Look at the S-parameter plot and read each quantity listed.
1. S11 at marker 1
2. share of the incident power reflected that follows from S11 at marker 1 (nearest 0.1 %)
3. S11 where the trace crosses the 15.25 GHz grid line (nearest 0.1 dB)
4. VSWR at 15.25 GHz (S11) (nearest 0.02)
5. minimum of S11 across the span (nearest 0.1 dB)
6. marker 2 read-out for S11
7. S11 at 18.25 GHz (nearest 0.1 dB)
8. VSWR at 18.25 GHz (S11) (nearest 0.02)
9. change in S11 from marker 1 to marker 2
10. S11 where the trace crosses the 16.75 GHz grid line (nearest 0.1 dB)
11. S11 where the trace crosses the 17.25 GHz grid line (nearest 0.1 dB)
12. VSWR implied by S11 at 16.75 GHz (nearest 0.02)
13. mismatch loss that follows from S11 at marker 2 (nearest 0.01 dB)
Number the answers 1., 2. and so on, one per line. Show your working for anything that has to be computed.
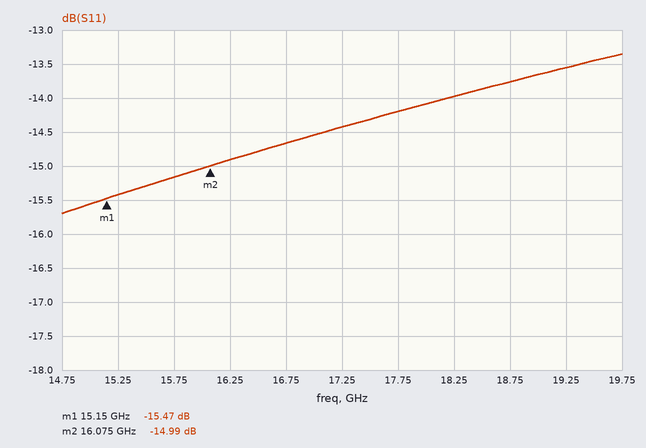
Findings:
1. -15.47 dB
2. 10^(-15.47/10) ≈ 2.8 %
3. -15.4 dB
4. |Γ| = 10^(-15.4/20) = 0.1698; VSWR = (1 + 0.1698)/(1 − 0.1698) ≈ 1.41, so 1.40 to the nearest 0.02
5. -15.7 dB
6. -14.99 dB
7. -14.0 dB
8. |Γ| = 10^(-14/20) = 0.1995; VSWR = (1 + 0.1995)/(1 − 0.1995) ≈ 1.50
9. -14.99 − (-15.47) = 0.48 dB
10. -14.7 dB
11. -14.4 dB
12. |Γ| = 10^(-14.7/20) = 0.1841; VSWR = (1 + 0.1841)/(1 − 0.1841) ≈ 1.45, so 1.46 to the nearest 0.02
13. −10 log10(1 − 10^(-14.99/10)) ≈ 0.14 dB
